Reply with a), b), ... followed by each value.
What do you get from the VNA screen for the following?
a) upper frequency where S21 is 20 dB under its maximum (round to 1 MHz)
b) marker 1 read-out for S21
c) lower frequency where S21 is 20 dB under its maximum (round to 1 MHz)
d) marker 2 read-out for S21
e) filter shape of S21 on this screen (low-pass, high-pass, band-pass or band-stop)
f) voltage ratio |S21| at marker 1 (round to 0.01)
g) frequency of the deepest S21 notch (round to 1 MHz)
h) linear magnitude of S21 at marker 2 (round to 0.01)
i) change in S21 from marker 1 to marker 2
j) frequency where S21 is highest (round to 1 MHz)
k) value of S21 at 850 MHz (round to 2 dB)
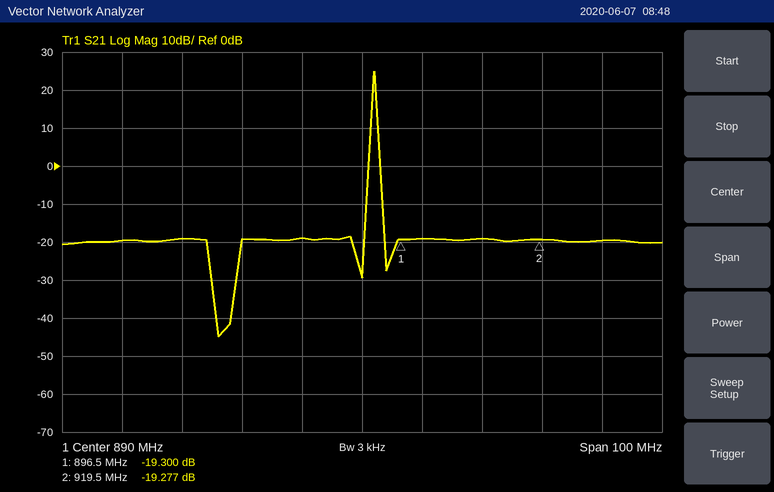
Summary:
a) 893 MHz
b) -19.300 dB
c) 891 MHz
d) -19.277 dB
e) band-pass
f) 0.11
g) 866 MHz
h) 0.11
i) 0.023 dB
j) 892 MHz
k) -20 dB
